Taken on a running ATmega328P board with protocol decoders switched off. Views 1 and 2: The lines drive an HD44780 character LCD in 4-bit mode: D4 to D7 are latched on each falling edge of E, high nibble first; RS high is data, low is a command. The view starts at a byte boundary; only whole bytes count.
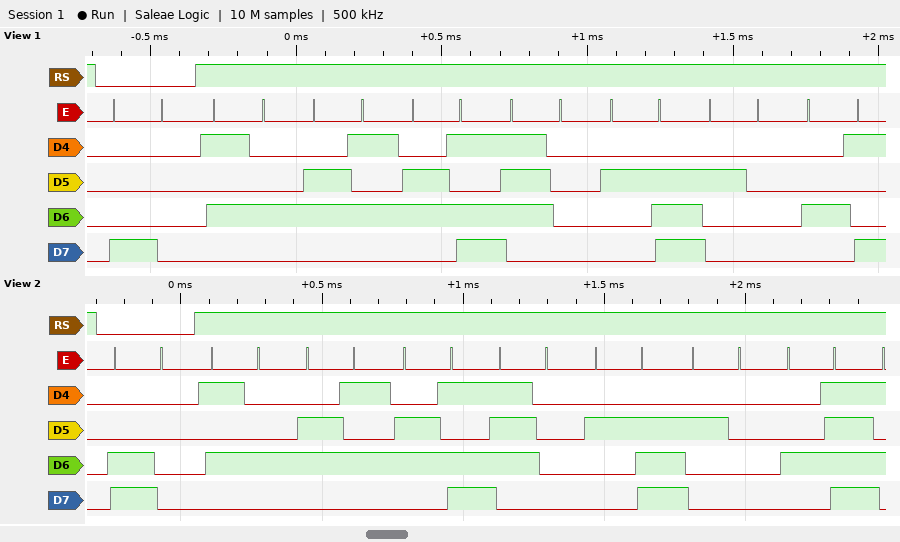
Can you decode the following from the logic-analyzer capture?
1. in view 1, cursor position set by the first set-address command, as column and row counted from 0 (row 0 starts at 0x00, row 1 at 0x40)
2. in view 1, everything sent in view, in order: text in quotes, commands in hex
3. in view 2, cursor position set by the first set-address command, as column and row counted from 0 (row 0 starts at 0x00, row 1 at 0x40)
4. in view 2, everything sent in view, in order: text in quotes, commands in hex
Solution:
column 0, row 0
0x80 "Temp. I"
column 0, row 1
0xC0 "Temp. O"
